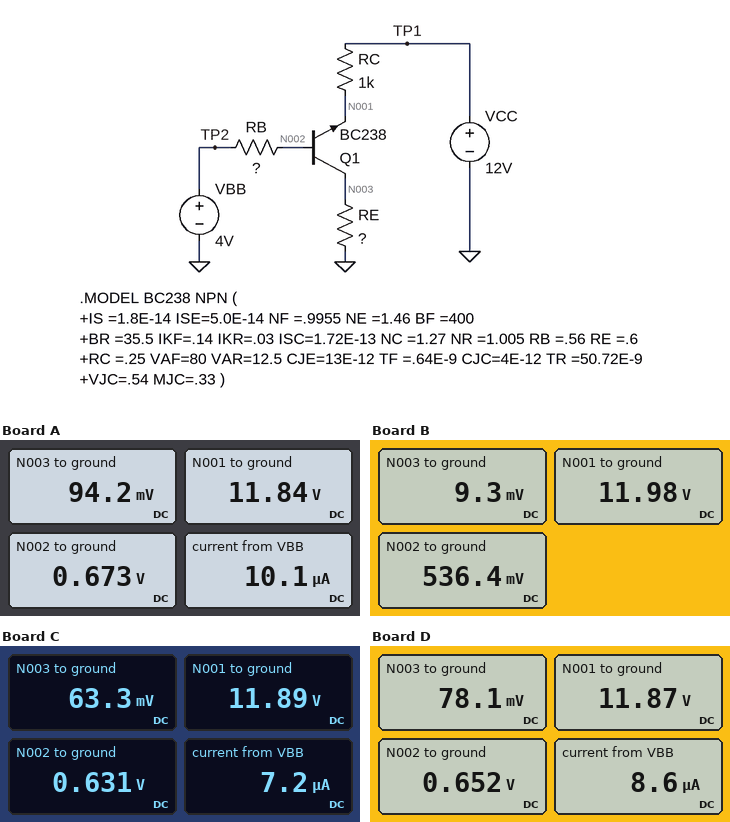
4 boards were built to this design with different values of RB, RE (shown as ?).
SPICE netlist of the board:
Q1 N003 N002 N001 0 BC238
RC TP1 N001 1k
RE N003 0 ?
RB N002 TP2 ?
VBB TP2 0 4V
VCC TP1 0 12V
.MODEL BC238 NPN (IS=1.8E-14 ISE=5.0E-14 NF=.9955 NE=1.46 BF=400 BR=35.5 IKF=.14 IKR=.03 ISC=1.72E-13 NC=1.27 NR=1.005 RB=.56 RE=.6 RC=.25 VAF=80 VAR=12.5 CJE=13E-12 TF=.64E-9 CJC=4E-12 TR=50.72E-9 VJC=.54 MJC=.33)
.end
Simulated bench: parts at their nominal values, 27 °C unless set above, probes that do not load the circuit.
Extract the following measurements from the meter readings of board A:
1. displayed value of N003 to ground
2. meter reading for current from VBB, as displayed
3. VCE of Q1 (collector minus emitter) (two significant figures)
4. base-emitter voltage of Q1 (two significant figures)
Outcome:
94.2 mV
10.1 µA
-12 V
-11 V
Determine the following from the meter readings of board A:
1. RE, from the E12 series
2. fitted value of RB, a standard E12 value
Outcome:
560 Ω
330 kΩ
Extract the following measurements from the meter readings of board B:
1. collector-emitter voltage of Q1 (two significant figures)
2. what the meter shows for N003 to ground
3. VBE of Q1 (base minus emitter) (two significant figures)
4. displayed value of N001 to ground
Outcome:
-12 V
9.3 mV
-11 V
11.98 V
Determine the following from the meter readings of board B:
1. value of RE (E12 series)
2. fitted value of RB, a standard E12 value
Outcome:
390 Ω
1.8 MΩ
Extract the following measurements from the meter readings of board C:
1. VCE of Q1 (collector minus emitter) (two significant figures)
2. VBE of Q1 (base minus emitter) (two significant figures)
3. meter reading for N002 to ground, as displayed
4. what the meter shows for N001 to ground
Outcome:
-12 V
-11 V
0.631 V
11.89 V
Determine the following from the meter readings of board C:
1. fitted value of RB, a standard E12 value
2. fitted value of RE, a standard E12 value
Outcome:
470 kΩ
560 Ω
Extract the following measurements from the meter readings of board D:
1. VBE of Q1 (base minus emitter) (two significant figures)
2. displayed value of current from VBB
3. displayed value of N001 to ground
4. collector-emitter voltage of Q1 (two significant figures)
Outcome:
-11 V
8.6 µA
11.87 V
-12 V
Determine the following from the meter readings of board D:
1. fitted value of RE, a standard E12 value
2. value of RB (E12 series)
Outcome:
560 Ω
390 kΩ
